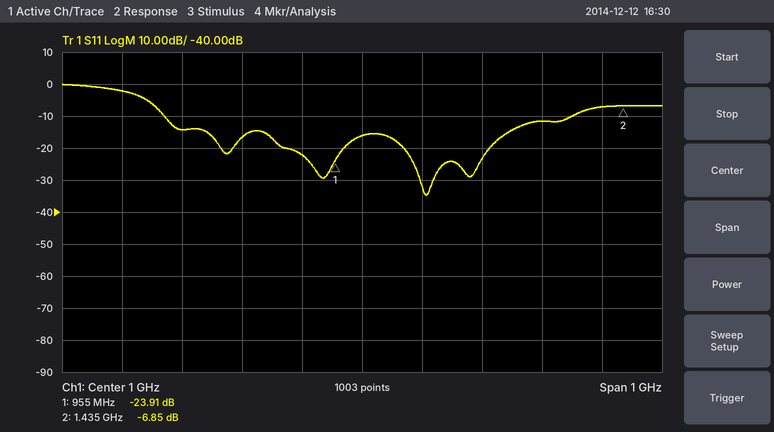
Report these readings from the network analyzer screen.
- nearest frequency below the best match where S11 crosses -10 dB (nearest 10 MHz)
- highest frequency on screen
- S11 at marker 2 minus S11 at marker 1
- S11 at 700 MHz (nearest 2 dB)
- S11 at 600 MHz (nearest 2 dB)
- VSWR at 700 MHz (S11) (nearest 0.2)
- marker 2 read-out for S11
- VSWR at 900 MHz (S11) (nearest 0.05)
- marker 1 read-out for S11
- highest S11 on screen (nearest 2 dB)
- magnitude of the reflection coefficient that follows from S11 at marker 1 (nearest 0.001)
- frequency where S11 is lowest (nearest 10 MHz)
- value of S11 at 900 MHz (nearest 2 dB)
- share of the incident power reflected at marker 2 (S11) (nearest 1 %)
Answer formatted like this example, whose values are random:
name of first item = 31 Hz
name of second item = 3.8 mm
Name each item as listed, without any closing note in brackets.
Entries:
nearest frequency below the best match where S11 crosses -10 dB = 670 MHz
highest frequency on screen = 1.5 GHz
S11 at marker 2 minus S11 at marker 1 = 17.06 dB
S11 at 700 MHz = -14 dB
S11 at 600 MHz = -2 dB
VSWR at 700 MHz (S11) = 1.4
marker 2 read-out for S11 = -6.85 dB
VSWR at 900 MHz (S11) = 1.15
marker 1 read-out for S11 = -23.91 dB
highest S11 on screen = 0 dB
magnitude of the reflection coefficient that follows from S11 at marker 1 = 0.064
frequency where S11 is lowest = 1.11 GHz
value of S11 at 900 MHz = -22 dB
share of the incident power reflected at marker 2 (S11) = 21 %
